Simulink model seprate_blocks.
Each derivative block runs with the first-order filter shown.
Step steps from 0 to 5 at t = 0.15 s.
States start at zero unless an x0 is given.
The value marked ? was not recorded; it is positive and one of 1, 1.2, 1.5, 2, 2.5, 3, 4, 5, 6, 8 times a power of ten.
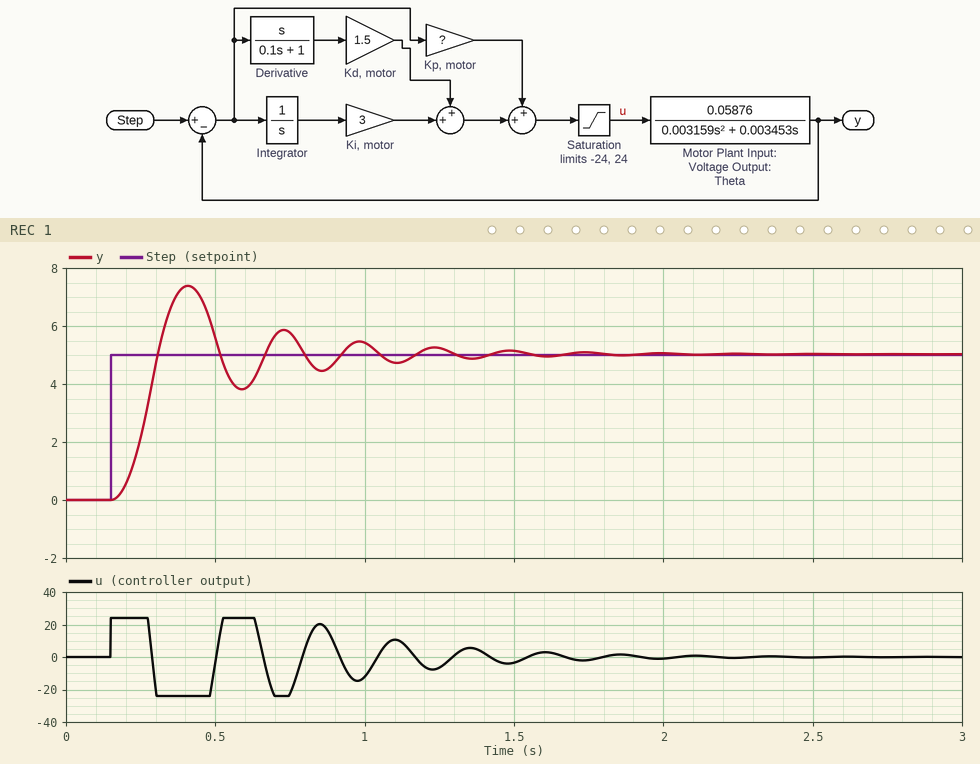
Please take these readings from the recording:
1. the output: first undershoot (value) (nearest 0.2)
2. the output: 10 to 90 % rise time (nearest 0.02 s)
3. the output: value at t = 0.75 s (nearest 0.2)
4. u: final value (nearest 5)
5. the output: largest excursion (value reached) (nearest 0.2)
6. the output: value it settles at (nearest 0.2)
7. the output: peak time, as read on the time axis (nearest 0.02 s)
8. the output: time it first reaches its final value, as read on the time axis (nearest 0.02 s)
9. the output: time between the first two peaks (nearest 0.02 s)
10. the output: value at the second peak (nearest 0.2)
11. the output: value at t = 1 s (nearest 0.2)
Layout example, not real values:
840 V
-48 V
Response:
3.8
0.10 s
5.8
0
7.4
5.0
0.40 s
0.30 s
0.32 s
5.8
5.4
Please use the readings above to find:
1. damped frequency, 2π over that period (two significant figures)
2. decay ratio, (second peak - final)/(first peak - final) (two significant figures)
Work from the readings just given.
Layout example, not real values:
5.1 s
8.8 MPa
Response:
20 rad/s
0.33
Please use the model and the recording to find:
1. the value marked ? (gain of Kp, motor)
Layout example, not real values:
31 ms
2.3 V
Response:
20
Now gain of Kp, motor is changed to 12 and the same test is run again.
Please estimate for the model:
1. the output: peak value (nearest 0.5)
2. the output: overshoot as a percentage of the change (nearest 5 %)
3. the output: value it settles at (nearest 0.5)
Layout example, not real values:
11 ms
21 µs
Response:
7.0
35 %
5.0
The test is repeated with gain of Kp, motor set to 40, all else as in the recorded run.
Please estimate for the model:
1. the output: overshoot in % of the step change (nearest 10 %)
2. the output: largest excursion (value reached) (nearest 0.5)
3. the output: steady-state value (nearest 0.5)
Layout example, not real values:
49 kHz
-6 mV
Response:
60 %
8.0
5.0
